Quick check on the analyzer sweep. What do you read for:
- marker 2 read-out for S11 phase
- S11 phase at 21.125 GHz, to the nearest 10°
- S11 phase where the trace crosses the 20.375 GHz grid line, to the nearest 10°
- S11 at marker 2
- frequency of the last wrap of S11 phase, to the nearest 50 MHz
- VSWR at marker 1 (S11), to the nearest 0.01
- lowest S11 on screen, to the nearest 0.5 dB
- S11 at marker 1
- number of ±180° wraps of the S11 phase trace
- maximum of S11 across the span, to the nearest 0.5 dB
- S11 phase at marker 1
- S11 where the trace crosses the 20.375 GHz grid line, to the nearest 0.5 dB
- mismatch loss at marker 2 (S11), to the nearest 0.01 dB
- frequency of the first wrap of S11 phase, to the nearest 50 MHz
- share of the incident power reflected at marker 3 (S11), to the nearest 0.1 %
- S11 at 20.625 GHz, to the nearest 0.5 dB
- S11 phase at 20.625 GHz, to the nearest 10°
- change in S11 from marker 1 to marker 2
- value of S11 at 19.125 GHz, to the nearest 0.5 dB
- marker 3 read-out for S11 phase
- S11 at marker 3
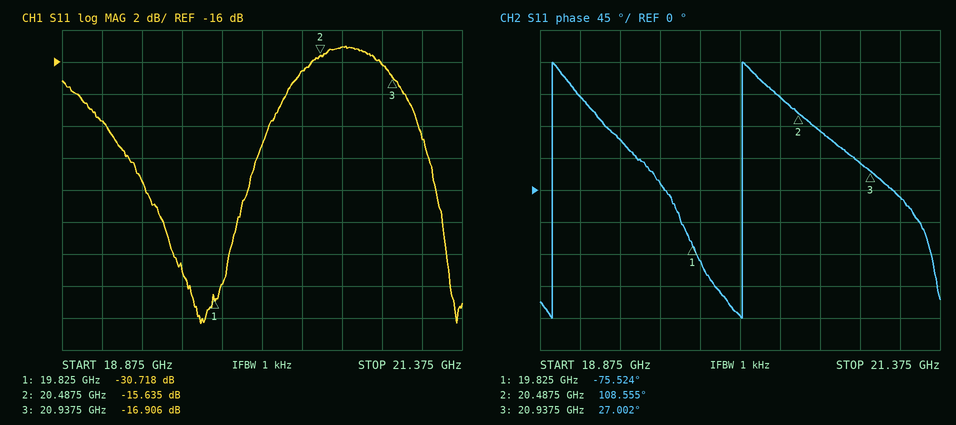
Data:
108.555°
-10°
130°
-15.635 dB
20.15 GHz
1.06
-32.5 dB
-30.718 dB
2
-15.0 dB
-75.524°
-16.5 dB
0.12 dB
18.95 GHz
2.0 %
-15.0 dB
80°
15.083 dB
-19.5 dB
27.002°
-16.906 dB
